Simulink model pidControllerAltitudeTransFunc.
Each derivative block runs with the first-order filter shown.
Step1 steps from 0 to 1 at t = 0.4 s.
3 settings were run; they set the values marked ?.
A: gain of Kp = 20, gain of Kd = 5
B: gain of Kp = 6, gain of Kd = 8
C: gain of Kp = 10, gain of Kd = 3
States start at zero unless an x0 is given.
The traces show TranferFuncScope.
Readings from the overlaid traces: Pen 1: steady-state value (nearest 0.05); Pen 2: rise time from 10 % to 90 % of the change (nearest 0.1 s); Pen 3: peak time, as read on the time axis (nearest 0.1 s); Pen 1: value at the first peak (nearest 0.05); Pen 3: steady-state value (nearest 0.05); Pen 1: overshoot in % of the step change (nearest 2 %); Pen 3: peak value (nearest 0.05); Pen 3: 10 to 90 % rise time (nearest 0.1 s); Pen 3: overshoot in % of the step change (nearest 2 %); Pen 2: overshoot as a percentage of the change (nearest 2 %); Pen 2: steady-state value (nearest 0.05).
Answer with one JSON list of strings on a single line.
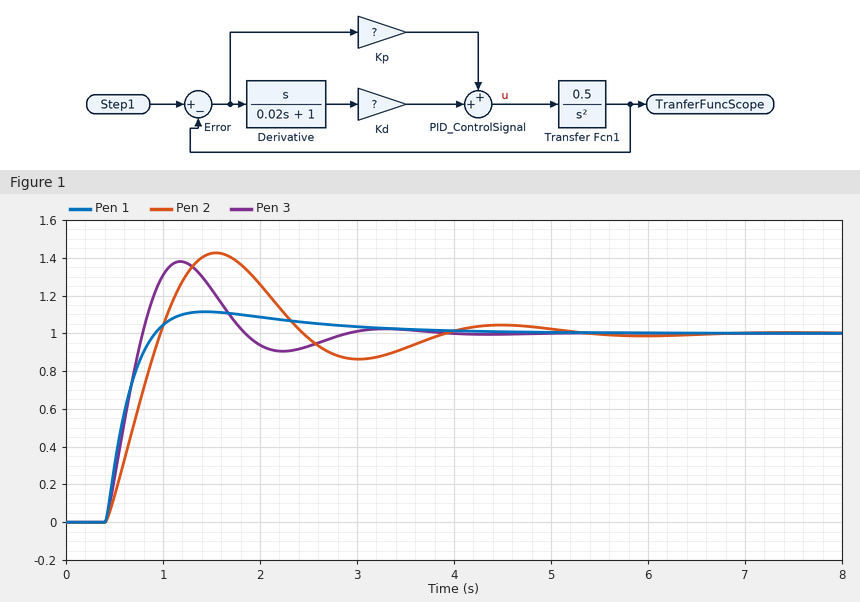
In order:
["1.00", "0.4 s", "1.2 s", "1.10", "1.00", "12 %", "1.40", "0.3 s", "38 %", "42 %", "1.00"]
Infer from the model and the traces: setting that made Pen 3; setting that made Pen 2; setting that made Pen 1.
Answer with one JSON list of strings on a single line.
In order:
["A", "C", "B"]
